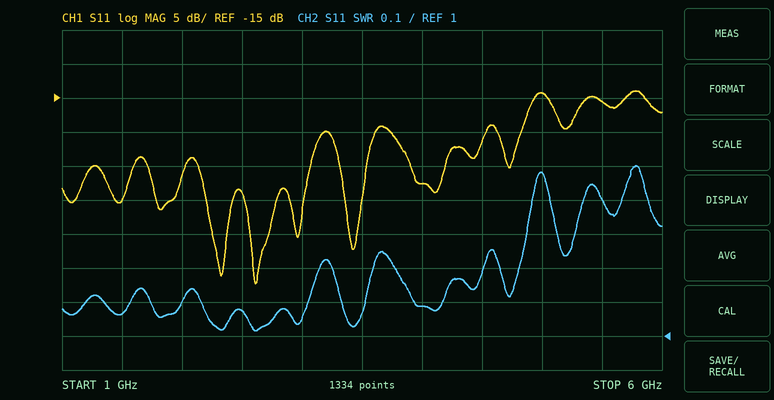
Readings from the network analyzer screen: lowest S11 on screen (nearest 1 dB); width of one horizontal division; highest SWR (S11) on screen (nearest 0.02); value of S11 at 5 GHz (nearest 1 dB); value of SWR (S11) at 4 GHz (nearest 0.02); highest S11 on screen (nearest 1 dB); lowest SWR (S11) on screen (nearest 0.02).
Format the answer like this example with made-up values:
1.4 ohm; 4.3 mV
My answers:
-42 dB; 500 MHz; 1.50; -14 dB; 1.08; -14 dB; 1.02
